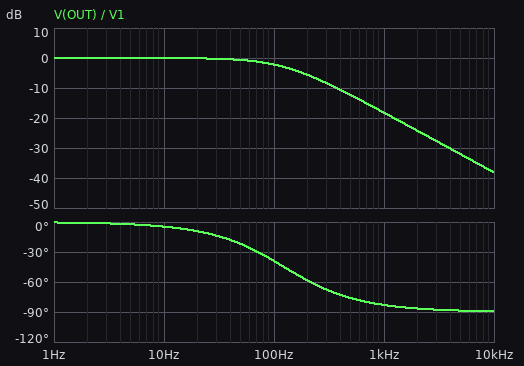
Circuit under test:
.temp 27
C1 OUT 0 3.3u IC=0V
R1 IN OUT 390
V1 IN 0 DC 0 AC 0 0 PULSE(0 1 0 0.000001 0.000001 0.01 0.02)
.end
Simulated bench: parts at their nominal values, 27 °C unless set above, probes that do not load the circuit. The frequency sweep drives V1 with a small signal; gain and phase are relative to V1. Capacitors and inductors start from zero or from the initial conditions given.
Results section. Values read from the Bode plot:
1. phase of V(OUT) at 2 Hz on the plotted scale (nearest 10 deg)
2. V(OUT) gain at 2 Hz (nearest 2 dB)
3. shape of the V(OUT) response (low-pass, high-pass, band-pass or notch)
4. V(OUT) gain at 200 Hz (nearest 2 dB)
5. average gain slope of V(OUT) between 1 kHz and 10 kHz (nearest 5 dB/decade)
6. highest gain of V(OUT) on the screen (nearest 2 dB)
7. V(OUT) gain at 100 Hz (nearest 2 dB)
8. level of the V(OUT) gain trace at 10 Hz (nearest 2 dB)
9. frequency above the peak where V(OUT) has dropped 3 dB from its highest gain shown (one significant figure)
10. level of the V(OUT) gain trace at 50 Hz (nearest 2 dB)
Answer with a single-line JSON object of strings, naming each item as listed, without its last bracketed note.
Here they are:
{"phase of V(OUT) at 2 Hz on the plotted scale": "0 deg", "V(OUT) gain at 2 Hz": "0 dB", "shape of the V(OUT) response": "low-pass", "V(OUT) gain at 200 Hz": "-6 dB", "average gain slope of V(OUT) between 1 kHz and 10 kHz": "-20 dB/decade", "highest gain of V(OUT) on the screen": "0 dB", "V(OUT) gain at 100 Hz": "-2 dB", "level of the V(OUT) gain trace at 10 Hz": "0 dB", "frequency above the peak where V(OUT) has dropped 3 dB from its highest gain shown": "100 Hz", "level of the V(OUT) gain trace at 50 Hz": "0 dB"}
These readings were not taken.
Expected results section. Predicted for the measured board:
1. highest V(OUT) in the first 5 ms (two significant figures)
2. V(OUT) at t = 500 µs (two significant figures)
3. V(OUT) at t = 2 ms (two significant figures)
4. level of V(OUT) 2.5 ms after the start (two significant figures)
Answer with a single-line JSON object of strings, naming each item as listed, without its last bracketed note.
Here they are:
{"highest V(OUT) in the first 5 ms": "980 mV", "V(OUT) at t = 500 µs": "320 mV", "V(OUT) at t = 2 ms": "790 mV", "level of V(OUT) 2.5 ms after the start": "860 mV"}
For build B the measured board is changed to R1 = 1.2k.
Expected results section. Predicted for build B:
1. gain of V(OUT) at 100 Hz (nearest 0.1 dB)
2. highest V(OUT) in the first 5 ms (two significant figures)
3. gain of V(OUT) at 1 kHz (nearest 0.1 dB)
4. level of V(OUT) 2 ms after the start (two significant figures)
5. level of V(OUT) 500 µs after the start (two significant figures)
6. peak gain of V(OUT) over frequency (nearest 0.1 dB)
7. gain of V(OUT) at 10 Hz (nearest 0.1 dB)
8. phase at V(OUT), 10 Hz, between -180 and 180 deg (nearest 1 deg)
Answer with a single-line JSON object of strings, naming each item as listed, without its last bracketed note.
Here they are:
{"gain of V(OUT) at 100 Hz": "-8.6 dB", "highest V(OUT) in the first 5 ms": "720 mV", "gain of V(OUT) at 1 kHz": "-27.9 dB", "level of V(OUT) 2 ms after the start": "400 mV", "level of V(OUT) 500 µs after the start": "120 mV", "peak gain of V(OUT) over frequency": "0 dB", "gain of V(OUT) at 10 Hz": "-0.3 dB", "phase at V(OUT), 10 Hz, between -180 and 180 deg": "-14 deg"}
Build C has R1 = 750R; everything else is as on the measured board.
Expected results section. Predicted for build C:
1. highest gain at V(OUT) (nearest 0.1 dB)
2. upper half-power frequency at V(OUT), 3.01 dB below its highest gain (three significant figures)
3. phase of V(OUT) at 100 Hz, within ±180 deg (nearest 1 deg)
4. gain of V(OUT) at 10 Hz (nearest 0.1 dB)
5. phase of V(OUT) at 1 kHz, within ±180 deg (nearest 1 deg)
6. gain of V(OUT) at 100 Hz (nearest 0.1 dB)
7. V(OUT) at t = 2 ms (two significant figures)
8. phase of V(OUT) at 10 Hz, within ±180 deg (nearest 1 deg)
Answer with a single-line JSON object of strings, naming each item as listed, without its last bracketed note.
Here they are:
{"highest gain at V(OUT)": "0 dB", "upper half-power frequency at V(OUT), 3.01 dB below its highest gain": "64.3 Hz", "phase of V(OUT) at 100 Hz, within ±180 deg": "-57 deg", "gain of V(OUT) at 10 Hz": "-0.1 dB", "phase of V(OUT) at 1 kHz, within ±180 deg": "-86 deg", "gain of V(OUT) at 100 Hz": "-5.3 dB", "V(OUT) at t = 2 ms": "550 mV", "phase of V(OUT) at 10 Hz, within ±180 deg": "-9 deg"}
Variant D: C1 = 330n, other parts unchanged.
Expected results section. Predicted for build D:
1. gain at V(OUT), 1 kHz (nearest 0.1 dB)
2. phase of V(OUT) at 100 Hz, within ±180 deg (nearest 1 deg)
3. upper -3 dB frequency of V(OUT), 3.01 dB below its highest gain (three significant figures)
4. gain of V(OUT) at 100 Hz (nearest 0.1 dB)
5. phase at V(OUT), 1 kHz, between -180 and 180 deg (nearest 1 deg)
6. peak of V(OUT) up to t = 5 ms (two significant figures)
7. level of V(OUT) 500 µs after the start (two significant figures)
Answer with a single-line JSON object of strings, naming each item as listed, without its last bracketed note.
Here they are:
{"gain at V(OUT), 1 kHz": "-2.2 dB", "phase of V(OUT) at 100 Hz, within ±180 deg": "-5 deg", "upper -3 dB frequency of V(OUT), 3.01 dB below its highest gain": "1.24 kHz", "gain of V(OUT) at 100 Hz": "0 dB", "phase at V(OUT), 1 kHz, between -180 and 180 deg": "-39 deg", "peak of V(OUT) up to t = 5 ms": "1.0 V", "level of V(OUT) 500 µs after the start": "980 mV"}
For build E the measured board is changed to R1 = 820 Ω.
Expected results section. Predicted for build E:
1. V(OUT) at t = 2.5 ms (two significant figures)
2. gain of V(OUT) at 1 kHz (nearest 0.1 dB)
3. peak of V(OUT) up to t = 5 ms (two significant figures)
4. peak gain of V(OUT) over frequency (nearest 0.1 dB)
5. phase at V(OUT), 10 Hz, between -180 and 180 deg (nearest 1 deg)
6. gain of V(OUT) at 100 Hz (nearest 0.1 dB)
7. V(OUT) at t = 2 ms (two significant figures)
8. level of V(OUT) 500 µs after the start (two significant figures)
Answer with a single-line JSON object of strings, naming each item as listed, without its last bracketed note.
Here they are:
{"V(OUT) at t = 2.5 ms": "600 mV", "gain of V(OUT) at 1 kHz": "-24.6 dB", "peak of V(OUT) up to t = 5 ms": "840 mV", "peak gain of V(OUT) over frequency": "0 dB", "phase at V(OUT), 10 Hz, between -180 and 180 deg": "-10 deg", "gain of V(OUT) at 100 Hz": "-5.9 dB", "V(OUT) at t = 2 ms": "520 mV", "level of V(OUT) 500 µs after the start": "170 mV"}
